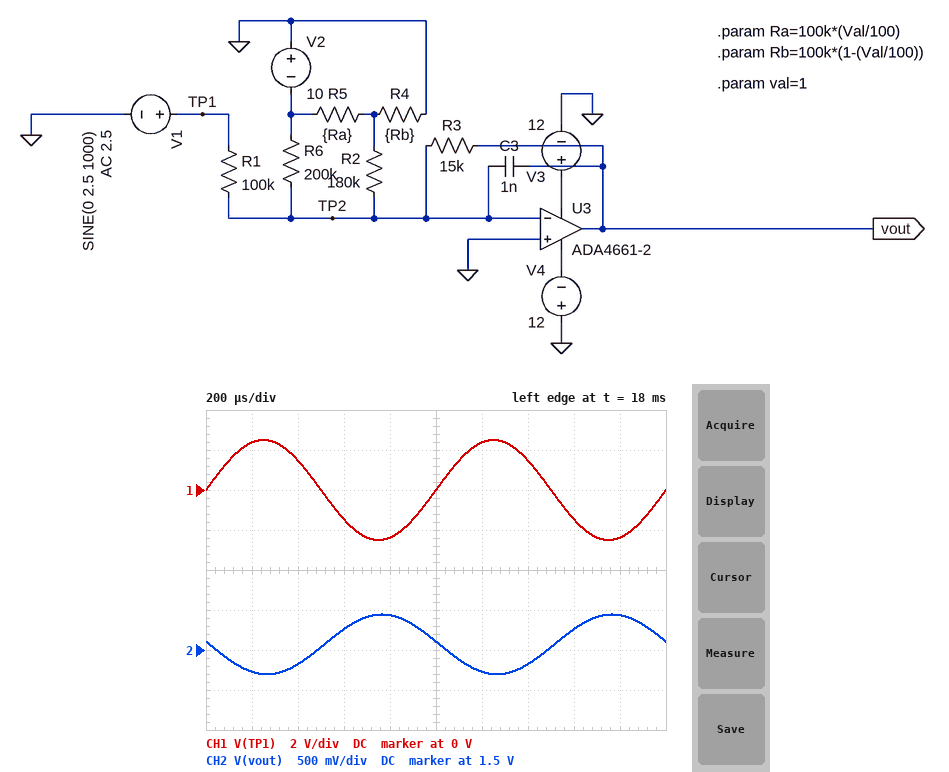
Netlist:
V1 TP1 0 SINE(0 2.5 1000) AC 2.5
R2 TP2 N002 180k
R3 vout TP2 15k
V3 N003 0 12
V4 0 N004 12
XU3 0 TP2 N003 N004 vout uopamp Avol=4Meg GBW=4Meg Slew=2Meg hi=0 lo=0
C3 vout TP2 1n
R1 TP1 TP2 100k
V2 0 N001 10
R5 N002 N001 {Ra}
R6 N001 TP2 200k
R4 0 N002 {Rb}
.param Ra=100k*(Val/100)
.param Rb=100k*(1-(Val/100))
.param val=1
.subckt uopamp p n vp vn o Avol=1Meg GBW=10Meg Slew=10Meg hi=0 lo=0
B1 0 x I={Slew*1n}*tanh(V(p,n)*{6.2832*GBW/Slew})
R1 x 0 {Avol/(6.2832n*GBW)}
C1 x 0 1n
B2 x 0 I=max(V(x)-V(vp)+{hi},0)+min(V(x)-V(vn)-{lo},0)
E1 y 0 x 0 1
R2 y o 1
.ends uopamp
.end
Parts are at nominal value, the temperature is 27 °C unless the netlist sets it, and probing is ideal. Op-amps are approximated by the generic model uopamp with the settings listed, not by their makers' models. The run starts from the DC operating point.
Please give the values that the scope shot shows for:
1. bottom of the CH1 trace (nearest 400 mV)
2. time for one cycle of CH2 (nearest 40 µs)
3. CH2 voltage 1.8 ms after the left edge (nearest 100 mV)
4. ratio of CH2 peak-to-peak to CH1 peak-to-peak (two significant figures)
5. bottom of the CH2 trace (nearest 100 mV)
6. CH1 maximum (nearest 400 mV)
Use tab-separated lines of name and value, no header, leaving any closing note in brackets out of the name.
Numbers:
bottom of the CH1 trace	-2.4 V
time for one cycle of CH2	1.00 ms
CH2 voltage 1.8 ms after the left edge	1.9 V
ratio of CH2 peak-to-peak to CH1 peak-to-peak	0.15
bottom of the CH2 trace	1.2 V
CH1 maximum	2.4 V
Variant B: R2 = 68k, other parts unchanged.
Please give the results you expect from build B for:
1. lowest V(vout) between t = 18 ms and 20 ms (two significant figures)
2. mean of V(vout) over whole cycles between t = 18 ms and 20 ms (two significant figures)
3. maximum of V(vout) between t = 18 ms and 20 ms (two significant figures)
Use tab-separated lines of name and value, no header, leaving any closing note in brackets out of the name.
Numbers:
lowest V(vout) between t = 18 ms and 20 ms	2.5 V
mean of V(vout) over whole cycles between t = 18 ms and 20 ms	2.9 V
maximum of V(vout) between t = 18 ms and 20 ms	3.3 V
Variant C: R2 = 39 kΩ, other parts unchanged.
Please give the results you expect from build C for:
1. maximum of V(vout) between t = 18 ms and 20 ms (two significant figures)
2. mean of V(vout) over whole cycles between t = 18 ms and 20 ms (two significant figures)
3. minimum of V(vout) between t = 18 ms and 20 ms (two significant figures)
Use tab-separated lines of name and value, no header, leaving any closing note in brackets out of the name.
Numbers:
maximum of V(vout) between t = 18 ms and 20 ms	4.8 V
mean of V(vout) over whole cycles between t = 18 ms and 20 ms	4.5 V
minimum of V(vout) between t = 18 ms and 20 ms	4.1 V
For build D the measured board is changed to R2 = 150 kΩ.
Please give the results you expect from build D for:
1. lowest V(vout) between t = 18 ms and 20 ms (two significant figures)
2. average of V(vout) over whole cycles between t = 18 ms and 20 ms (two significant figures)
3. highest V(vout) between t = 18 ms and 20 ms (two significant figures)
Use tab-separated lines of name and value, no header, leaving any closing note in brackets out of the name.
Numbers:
lowest V(vout) between t = 18 ms and 20 ms	1.4 V
average of V(vout) over whole cycles between t = 18 ms and 20 ms	1.7 V
highest V(vout) between t = 18 ms and 20 ms	2.1 V
